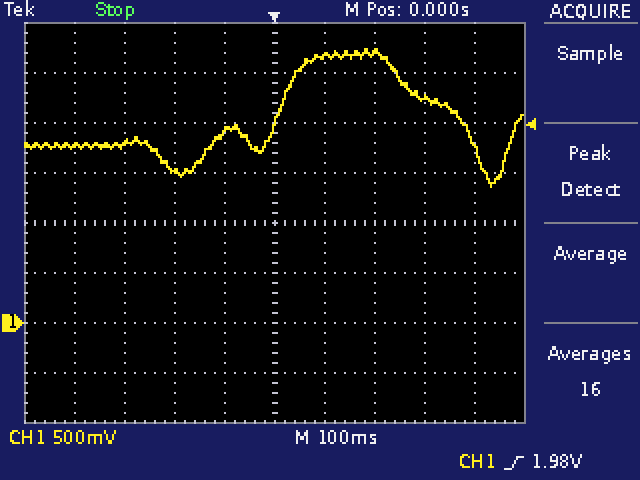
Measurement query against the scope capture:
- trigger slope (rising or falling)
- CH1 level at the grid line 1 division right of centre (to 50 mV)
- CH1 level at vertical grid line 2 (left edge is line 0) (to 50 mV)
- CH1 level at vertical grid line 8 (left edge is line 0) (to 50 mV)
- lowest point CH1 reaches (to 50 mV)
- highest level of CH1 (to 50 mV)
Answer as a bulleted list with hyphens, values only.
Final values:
- rising
- 2.65 V
- 1.80 V
- 2.25 V
- 1.35 V
- 2.75 V
